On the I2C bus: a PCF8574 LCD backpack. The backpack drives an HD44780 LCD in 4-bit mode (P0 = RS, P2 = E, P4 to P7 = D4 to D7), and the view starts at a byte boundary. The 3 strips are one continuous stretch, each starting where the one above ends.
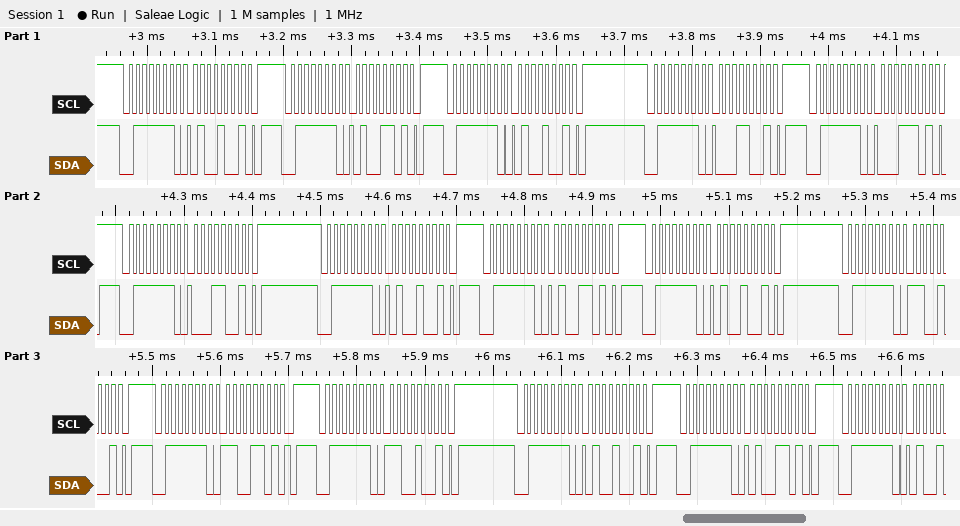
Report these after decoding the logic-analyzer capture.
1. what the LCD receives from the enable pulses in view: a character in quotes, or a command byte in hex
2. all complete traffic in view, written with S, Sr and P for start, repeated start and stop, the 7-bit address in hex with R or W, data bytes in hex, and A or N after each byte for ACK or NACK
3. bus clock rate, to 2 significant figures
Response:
'A' 'L'
S 3FW A 49 A P S 3FW A 4D A P S 3FW A 49 A P S 3FW A 19 A P S 3FW A 1D A P S 3FW A 19 A P S 3FW A 49 A P S 3FW A 4D A P S 3FW A 49 A P S 3FW A C9 A P S 3FW A CD A P S 3FW A C9 A P S 3FW A 49 A P S 3FW A 4D A P S 3FW A
100 kHz
